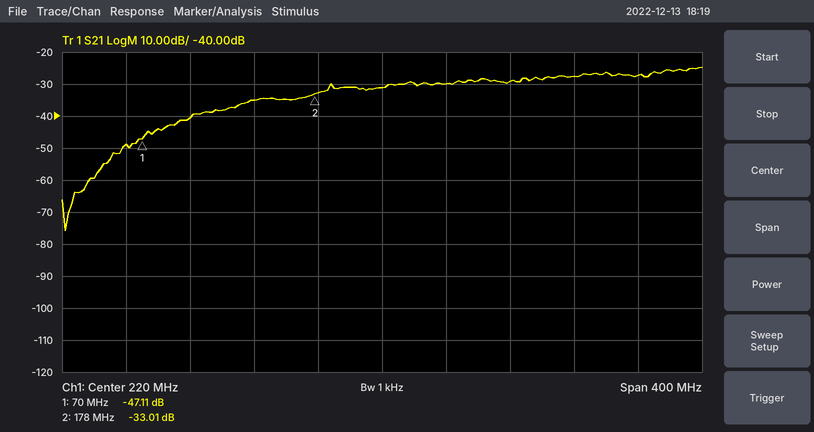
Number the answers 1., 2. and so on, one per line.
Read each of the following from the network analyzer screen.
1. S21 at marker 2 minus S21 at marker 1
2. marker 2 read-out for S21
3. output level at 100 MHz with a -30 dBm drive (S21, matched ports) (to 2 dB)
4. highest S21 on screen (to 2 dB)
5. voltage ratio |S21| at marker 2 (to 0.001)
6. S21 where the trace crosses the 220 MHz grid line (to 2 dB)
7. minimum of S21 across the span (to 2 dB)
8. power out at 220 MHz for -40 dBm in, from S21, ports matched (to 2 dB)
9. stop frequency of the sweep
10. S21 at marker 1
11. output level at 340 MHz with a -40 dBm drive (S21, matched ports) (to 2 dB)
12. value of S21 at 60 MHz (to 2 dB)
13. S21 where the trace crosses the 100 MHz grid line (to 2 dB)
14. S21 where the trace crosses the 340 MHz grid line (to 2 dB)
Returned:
1. 14.10 dB
2. -33.01 dB
3. -70 dBm
4. -24 dB
5. 0.022
6. -32 dB
7. -76 dB
8. -72 dBm
9. 420 MHz
10. -47.11 dB
11. -68 dBm
12. -48 dB
13. -40 dB
14. -28 dB
